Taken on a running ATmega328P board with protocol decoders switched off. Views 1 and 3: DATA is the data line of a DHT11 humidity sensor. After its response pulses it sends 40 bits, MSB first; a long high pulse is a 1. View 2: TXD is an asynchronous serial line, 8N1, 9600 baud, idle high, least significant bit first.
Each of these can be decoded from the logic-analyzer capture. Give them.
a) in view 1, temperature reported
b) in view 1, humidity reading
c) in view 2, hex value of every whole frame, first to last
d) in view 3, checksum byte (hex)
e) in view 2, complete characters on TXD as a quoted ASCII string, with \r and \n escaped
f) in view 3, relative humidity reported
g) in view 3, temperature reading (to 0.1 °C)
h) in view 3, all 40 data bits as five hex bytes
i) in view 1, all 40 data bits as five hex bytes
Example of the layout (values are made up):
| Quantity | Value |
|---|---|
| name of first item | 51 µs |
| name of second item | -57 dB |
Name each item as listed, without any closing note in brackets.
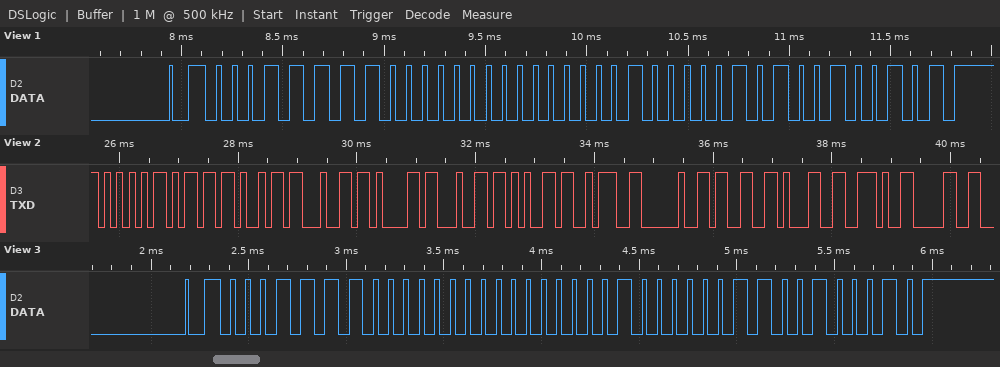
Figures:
| Quantity | Value |
|---|---|
| in view 1, temperature reported | 1.5 °C |
| in view 1, humidity reading | 31 % |
| in view 2, hex value of every whole frame, first to last | 0x55 0x6D 0x69 0x64 0x61 0x64 0x65 0x3A 0x20 0x33 0x31 0x2E 0x30 |
| in view 3, checksum byte | 0x22 |
| in view 2, complete characters on TXD as a quoted ASCII string, with \r and \n escaped | "Umidade: 31.0" |
| in view 3, relative humidity reported | 30 % |
| in view 3, temperature reading | 1.3 °C |
| in view 3, all 40 data bits as five hex bytes | 1E 00 01 03 22 |
| in view 1, all 40 data bits as five hex bytes | 1F 00 01 05 25 |
